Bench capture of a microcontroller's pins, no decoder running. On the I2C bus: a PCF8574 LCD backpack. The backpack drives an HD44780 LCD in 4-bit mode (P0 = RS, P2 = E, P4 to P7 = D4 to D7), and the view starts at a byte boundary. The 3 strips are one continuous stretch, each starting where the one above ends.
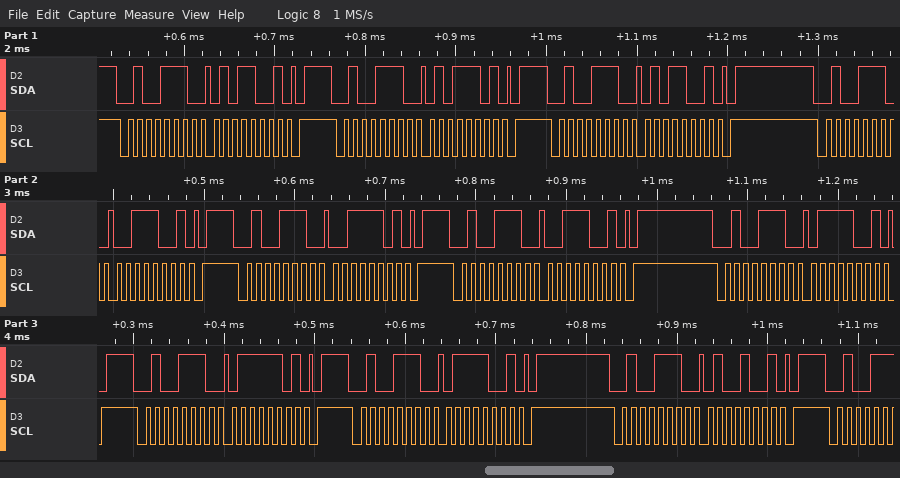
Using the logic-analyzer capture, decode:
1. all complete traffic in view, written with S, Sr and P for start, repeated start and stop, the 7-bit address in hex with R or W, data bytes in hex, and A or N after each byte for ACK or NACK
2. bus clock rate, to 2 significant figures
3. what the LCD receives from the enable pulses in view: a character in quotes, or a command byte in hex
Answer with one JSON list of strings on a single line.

["S 27W A 59 A P S 27W A 5D A P S 27W A 59 A P S 27W A 39 A P S 27W A 3D A P S 27W A 39 A P S 27W A 79 A P S 27W A 7D A P S 27W A 79 A P S 27W A 49 A P", "100 kHz", "'S'"]
